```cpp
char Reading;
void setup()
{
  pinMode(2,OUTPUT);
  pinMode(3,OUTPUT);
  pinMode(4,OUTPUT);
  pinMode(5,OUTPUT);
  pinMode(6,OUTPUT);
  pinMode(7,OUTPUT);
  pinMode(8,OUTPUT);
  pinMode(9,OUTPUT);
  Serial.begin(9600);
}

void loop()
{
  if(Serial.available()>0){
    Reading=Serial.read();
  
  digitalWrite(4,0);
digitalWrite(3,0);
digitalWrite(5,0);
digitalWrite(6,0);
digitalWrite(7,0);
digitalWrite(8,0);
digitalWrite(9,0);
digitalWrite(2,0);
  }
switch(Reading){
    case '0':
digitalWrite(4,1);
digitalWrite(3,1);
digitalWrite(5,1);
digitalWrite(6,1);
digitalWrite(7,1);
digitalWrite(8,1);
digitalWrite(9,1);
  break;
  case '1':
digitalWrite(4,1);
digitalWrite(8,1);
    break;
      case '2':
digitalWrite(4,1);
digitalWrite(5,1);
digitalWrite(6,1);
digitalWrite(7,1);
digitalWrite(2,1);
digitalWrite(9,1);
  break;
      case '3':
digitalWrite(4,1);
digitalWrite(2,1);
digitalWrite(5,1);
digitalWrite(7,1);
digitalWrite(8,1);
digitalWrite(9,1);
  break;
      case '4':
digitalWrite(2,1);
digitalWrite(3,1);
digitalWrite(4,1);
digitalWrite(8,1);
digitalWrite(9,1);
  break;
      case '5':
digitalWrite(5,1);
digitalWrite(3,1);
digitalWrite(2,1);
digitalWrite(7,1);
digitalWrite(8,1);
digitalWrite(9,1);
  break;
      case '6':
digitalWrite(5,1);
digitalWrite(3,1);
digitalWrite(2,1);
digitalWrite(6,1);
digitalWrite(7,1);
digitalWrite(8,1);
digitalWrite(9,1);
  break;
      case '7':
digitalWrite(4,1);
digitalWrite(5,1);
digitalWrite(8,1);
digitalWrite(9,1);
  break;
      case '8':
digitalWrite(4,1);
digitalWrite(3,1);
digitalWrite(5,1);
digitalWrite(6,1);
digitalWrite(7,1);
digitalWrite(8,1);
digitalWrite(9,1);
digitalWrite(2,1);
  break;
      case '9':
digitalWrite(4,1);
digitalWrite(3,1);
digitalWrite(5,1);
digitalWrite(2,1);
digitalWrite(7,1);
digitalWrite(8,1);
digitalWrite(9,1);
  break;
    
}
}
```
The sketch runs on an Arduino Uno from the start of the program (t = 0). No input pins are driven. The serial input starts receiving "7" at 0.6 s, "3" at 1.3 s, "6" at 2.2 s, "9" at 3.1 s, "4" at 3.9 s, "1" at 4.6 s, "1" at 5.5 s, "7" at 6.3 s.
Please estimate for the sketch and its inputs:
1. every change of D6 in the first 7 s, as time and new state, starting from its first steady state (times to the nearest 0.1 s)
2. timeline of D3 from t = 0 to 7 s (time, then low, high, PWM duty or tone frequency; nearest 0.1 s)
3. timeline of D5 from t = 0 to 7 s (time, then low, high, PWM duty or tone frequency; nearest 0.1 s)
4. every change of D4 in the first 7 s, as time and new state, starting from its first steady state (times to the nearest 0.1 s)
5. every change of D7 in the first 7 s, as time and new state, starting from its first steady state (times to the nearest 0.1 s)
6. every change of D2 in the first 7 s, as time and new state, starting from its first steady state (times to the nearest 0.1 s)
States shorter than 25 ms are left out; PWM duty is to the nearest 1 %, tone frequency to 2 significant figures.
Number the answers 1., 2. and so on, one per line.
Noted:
1. 0 s low; 2.2 s high; 3.1 s low
2. 0 s low; 2.2 s high; 4.6 s low
3. 0 s low; 0.6 s high; 3.9 s low; 6.3 s high
4. 0 s low; 0.6 s high; 2.2 s low; 3.1 s high
5. 0 s low; 1.3 s high; 3.9 s low
6. 0 s low; 1.3 s high; 4.6 s low
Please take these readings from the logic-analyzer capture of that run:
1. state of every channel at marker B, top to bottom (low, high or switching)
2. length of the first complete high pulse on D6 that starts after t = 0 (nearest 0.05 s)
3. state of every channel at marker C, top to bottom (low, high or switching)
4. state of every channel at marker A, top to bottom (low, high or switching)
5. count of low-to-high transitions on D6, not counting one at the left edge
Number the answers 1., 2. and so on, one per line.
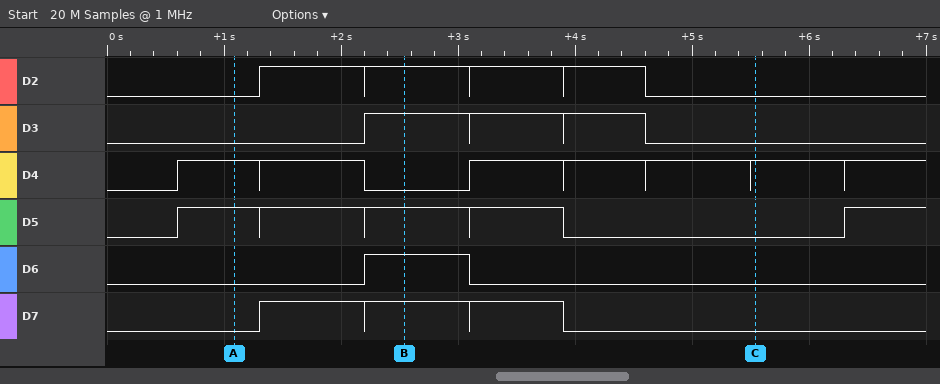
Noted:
1. D2 high, D3 high, D4 low, D5 high, D6 high, D7 high
2. 0.90 s
3. D2 low, D3 low, D4 high, D5 low, D6 low, D7 low
4. D2 low, D3 low, D4 high, D5 high, D6 low, D7 low
5. 1
